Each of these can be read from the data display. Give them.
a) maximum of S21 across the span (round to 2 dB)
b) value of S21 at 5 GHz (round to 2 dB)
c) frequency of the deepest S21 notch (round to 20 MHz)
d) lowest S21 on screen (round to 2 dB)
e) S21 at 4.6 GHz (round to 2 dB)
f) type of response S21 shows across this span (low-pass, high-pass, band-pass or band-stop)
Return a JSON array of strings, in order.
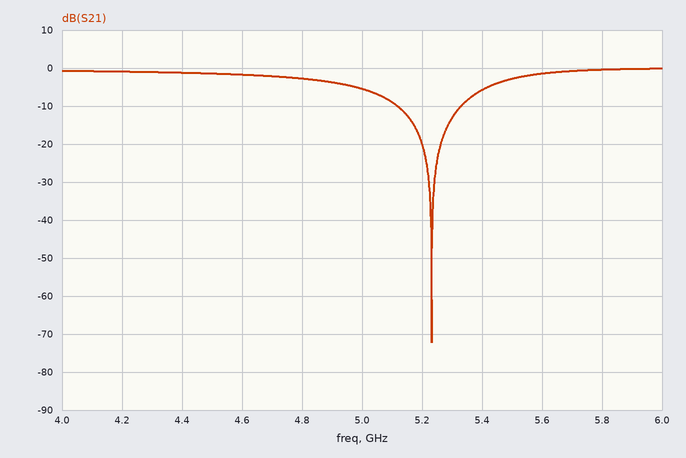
["0 dB", "-6 dB", "5.24 GHz", "-72 dB", "-2 dB", "band-stop"]
